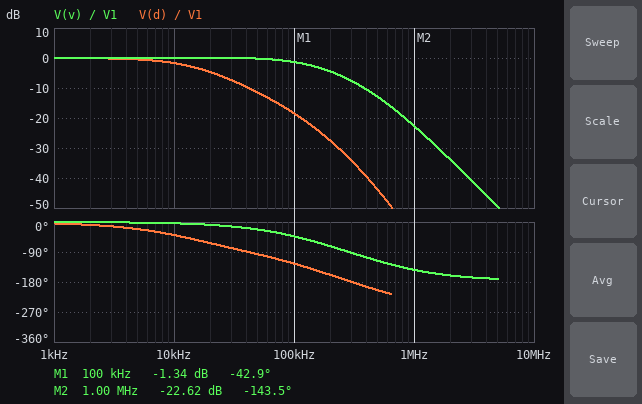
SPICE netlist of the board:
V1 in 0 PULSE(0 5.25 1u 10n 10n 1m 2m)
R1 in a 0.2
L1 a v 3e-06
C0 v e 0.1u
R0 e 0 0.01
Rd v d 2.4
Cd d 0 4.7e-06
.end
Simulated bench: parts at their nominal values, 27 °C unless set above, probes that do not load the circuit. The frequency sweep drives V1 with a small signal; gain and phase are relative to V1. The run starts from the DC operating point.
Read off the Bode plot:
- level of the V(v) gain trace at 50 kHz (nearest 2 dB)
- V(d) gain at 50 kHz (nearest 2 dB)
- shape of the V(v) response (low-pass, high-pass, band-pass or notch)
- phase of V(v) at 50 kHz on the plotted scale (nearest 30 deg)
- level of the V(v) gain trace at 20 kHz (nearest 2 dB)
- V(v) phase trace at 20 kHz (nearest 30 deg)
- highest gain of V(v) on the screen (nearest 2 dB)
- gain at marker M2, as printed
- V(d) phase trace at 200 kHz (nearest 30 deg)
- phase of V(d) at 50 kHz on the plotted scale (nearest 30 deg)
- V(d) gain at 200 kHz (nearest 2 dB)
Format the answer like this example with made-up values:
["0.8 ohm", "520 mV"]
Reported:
["0 dB", "-12 dB", "low-pass", "-30 deg", "0 dB", "0 deg", "0 dB", "-22.62 dB", "-150 deg", "-90 deg", "-28 dB"]
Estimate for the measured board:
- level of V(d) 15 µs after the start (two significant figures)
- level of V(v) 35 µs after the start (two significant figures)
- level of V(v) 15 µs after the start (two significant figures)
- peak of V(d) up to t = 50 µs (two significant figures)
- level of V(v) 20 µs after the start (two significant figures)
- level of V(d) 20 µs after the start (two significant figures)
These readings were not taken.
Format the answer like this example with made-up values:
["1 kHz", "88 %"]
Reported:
["3.6 V", "5.3 V", "5.3 V", "5.2 V", "5.3 V", "4.2 V"]
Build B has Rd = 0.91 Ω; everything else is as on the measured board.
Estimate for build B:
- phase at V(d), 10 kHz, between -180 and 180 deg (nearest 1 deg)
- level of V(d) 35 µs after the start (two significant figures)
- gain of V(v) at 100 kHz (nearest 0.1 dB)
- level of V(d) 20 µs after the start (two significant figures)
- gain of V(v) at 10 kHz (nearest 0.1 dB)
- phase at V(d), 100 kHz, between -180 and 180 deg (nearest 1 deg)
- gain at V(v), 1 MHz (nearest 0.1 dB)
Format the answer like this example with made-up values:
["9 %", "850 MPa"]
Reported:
["-19 deg", "5.2 V", "-5.8 dB", "5.5 V", "0.3 dB", "-148 deg", "-27.5 dB"]
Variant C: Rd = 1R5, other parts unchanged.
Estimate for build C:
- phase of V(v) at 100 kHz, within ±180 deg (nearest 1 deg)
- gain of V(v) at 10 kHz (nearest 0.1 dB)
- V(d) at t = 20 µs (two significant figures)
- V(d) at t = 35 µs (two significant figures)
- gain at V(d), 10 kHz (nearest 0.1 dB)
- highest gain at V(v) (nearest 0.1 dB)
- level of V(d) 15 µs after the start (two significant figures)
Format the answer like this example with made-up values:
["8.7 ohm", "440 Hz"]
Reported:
["-59 deg", "0.2 dB", "5.0 V", "5.2 V", "-0.6 dB", "0.5 dB", "4.5 V"]
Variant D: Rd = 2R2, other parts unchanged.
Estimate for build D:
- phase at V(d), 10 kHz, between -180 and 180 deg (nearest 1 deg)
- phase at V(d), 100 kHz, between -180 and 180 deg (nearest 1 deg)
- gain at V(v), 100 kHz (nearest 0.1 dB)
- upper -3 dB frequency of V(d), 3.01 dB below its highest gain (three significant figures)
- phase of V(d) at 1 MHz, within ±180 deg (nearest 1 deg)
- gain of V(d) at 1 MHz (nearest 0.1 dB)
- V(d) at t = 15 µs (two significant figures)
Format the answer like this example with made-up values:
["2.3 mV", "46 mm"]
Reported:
["-37 deg", "-127 deg", "-1.6 dB", "15.9 kHz", "130 deg", "-59.2 dB", "3.8 V"]
